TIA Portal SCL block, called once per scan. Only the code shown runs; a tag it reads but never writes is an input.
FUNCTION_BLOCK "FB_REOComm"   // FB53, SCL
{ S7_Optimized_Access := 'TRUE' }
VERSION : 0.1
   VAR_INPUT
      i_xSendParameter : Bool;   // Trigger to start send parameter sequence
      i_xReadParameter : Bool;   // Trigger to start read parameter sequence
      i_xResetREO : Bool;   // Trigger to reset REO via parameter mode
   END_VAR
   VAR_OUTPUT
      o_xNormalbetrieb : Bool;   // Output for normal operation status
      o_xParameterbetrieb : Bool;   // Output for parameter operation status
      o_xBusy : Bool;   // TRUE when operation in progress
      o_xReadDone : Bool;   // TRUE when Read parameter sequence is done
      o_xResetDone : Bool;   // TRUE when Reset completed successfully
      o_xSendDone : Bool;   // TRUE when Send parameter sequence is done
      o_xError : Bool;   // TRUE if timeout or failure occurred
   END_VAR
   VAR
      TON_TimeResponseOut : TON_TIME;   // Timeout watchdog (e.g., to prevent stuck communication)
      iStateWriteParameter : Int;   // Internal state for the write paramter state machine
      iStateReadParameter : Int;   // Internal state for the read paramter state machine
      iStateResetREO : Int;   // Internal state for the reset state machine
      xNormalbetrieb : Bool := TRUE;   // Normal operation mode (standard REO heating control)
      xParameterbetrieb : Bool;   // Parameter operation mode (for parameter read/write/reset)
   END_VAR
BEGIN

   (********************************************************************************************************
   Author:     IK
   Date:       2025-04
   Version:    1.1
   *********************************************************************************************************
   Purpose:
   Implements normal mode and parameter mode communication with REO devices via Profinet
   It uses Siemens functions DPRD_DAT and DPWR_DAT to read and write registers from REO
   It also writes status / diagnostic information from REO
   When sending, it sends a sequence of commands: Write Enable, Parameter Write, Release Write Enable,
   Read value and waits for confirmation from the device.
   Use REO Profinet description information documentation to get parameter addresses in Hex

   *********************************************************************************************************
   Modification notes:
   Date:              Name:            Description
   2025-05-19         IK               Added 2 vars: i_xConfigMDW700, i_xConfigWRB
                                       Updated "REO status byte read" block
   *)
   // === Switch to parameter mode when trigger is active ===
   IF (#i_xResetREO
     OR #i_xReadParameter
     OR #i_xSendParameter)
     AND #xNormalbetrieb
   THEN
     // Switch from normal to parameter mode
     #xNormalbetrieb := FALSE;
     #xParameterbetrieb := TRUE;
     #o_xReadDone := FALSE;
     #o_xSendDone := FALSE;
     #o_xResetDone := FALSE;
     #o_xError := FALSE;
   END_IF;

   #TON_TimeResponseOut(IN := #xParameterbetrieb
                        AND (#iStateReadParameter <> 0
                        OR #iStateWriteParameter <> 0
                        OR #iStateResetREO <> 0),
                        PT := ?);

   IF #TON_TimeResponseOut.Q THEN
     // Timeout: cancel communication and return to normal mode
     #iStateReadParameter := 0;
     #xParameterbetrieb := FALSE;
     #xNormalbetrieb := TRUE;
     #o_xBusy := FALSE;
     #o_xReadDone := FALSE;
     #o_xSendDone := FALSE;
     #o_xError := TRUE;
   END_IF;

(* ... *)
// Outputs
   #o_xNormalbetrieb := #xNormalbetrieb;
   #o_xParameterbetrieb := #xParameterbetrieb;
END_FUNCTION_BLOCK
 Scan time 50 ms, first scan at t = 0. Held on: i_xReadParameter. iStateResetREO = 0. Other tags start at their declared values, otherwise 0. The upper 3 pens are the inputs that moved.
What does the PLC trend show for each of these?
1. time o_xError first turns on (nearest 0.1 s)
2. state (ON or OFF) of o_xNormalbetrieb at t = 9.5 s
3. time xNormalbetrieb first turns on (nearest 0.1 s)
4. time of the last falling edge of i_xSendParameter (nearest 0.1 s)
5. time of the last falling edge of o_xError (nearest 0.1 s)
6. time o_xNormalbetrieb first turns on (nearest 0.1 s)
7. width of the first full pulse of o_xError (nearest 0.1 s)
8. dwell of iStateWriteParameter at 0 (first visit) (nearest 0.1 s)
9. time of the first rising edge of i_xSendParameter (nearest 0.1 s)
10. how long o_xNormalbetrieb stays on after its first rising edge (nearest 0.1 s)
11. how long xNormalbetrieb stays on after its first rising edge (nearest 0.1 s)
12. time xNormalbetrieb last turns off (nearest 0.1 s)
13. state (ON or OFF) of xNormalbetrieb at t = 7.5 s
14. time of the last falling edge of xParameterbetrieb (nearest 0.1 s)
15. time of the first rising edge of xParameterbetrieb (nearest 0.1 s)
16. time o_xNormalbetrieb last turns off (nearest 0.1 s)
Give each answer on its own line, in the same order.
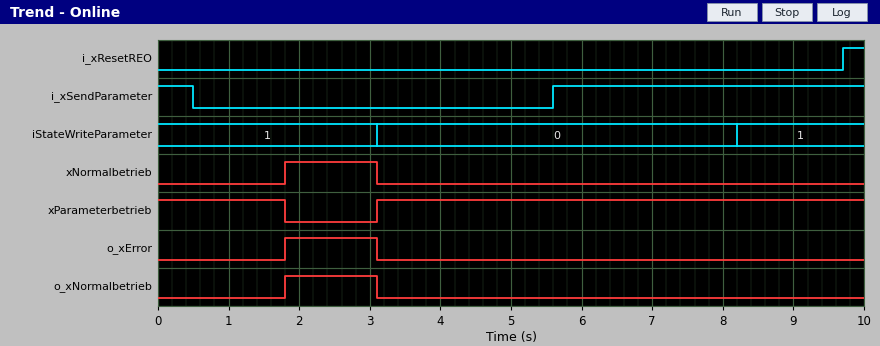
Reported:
1.8 s
OFF
1.8 s
0.5 s
3.1 s
1.8 s
1.3 s
5.1 s
5.6 s
1.3 s
1.3 s
3.1 s
OFF
1.8 s
3.1 s
3.1 s
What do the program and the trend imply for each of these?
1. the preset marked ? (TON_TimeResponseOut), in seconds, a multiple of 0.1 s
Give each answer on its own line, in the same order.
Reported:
1.8 s
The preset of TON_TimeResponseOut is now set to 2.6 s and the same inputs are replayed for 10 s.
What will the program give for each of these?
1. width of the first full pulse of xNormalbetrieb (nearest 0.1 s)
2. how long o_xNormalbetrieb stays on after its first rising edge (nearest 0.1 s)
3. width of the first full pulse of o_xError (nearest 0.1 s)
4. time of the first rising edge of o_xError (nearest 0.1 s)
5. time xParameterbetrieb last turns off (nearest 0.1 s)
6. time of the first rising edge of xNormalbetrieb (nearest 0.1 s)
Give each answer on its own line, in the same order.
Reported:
0.5 s
0.5 s
0.5 s
2.6 s
2.6 s
2.6 s
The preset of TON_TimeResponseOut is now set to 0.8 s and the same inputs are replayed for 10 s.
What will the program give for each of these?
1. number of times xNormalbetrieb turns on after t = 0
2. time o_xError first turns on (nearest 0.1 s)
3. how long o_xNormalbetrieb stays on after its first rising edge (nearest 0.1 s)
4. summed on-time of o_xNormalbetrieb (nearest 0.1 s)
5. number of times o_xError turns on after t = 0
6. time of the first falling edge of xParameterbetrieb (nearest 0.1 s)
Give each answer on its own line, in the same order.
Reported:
2
0.8 s
2.3 s
3.3 s
2
0.8 s
